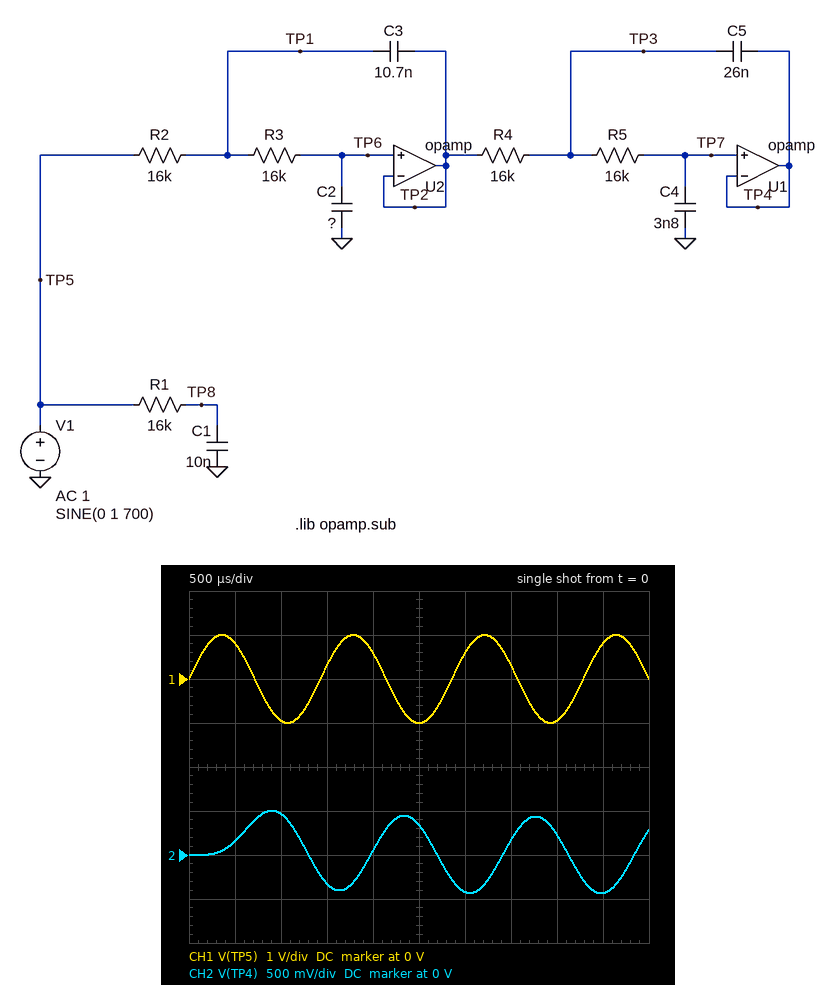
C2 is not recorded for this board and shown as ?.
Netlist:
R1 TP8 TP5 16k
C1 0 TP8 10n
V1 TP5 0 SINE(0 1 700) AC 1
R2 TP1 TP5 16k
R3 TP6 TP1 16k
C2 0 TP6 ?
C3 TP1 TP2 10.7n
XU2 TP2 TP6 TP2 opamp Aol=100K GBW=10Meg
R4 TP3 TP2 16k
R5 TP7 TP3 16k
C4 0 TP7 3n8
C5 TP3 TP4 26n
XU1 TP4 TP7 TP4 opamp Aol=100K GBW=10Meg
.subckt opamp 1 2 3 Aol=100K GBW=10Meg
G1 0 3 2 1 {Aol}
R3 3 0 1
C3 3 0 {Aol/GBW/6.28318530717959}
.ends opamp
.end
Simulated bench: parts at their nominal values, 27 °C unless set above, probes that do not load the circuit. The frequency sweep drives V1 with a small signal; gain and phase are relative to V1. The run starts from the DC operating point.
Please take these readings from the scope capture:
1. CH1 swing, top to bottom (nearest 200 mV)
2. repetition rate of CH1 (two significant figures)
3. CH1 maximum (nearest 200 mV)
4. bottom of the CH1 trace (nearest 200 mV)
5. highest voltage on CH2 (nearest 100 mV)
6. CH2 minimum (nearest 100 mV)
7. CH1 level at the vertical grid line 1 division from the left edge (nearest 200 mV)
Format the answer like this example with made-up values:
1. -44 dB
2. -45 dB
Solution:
1. 2.0 V
2. 700 Hz
3. 1.0 V
4. -1.0 V
5. 500 mV
6. -400 mV
7. 800 mV
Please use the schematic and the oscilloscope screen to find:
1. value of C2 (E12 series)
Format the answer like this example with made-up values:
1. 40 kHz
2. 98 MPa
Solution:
1. 22 nF
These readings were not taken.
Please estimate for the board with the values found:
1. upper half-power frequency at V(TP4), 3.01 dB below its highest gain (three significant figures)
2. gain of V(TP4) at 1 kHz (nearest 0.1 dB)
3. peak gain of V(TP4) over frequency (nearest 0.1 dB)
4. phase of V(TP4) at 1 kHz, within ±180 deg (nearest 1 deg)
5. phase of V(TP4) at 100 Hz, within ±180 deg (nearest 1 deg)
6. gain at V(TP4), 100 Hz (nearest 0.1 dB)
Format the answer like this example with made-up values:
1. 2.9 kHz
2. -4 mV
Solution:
1. 285 Hz
2. -11.0 dB
3. 0 dB
4. 163 deg
5. -29 deg
6. -0.5 dB
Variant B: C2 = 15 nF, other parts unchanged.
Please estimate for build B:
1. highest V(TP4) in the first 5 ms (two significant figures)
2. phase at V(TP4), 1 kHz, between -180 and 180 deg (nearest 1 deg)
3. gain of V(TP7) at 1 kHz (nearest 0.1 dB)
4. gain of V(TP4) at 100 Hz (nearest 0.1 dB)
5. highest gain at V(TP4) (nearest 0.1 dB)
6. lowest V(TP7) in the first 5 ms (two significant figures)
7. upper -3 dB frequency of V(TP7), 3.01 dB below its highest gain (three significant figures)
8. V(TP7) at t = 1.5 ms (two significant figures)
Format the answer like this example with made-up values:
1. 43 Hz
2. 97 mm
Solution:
1. 650 mV
2. 168 deg
3. -7.4 dB
4. -0.2 dB
5. 0 dB
6. -640 mV
7. 551 Hz
8. -560 mV
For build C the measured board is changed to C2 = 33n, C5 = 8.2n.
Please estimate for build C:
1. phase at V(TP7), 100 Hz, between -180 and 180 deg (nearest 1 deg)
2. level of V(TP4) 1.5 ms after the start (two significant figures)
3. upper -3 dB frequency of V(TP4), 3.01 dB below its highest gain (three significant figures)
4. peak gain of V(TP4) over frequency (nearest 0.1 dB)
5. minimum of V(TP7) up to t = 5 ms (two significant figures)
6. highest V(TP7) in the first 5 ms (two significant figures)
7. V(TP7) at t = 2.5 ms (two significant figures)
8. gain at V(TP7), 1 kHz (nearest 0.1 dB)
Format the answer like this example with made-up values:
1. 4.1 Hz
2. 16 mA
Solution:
1. -39 deg
2. -140 mV
3. 164 Hz
4. 0 dB
5. -210 mV
6. 330 mV
7. 160 mV
8. -17.3 dB
